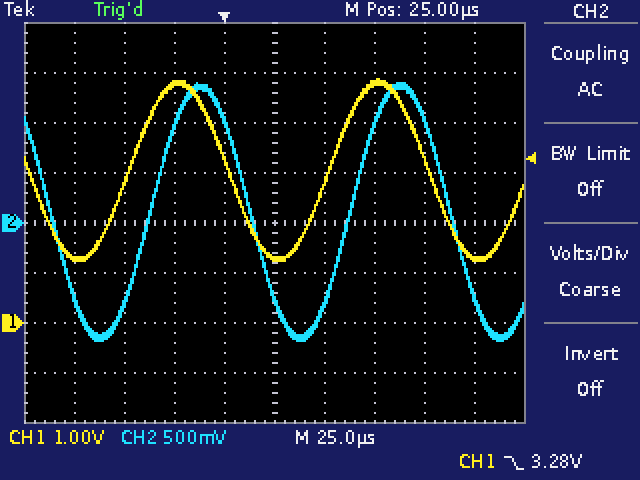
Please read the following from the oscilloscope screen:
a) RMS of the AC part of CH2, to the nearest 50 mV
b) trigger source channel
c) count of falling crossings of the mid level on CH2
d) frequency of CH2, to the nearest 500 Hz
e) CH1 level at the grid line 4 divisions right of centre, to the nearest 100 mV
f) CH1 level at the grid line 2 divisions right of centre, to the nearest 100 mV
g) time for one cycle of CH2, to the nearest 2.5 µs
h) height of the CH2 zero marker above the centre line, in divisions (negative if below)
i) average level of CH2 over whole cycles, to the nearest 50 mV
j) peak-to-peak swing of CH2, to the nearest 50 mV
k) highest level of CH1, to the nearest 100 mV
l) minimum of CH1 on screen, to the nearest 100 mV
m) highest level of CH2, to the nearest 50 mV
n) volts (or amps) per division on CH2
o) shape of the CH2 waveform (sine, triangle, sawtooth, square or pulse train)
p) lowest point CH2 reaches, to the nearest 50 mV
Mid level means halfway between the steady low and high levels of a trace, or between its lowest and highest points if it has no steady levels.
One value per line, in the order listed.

900 mV
CH1
3
10.0 kHz
1.3 V
4.8 V
100.0 µs
0.0 div
100 mV
2.60 V
4.9 V
1.2 V
1.40 V
500 mV
sine
-1.20 V
